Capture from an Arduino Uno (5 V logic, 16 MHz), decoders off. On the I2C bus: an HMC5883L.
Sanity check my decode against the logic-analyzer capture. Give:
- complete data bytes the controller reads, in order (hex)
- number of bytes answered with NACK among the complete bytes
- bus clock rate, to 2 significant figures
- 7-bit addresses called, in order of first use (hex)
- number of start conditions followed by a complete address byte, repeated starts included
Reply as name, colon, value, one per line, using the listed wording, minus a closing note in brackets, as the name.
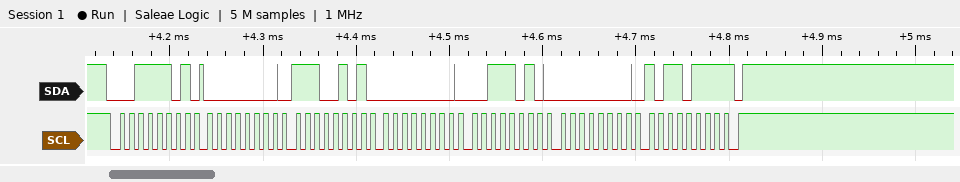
complete data bytes the controller reads, in order: 00 E5 00 3A 00 B7
number of bytes answered with NACK among the complete bytes: 1
bus clock rate, to 2 significant figures: 100 kHz
7-bit addresses called, in order of first use: 0x1E
number of start conditions followed by a complete address byte, repeated starts included: 1
